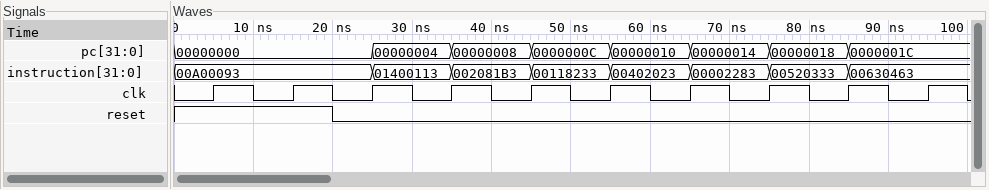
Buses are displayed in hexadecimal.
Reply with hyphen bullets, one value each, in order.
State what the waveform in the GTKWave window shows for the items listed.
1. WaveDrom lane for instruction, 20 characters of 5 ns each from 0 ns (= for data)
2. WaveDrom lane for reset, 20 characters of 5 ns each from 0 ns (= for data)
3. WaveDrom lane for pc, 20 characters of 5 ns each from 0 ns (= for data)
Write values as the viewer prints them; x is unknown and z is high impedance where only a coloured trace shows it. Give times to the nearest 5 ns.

- {name: 'instruction', wave: '=....=.=.=.=.=.=.=..', data: '00A00093 01400113 002081B3 00118233 00402023 00002283 00520333 00630463'}
- {name: 'reset', wave: '1...0...............'}
- {name: 'pc', wave: '=....=.=.=.=.=.=.=..', data: '00000000 00000004 00000008 0000000C 00000010 00000014 00000018 0000001C'}
